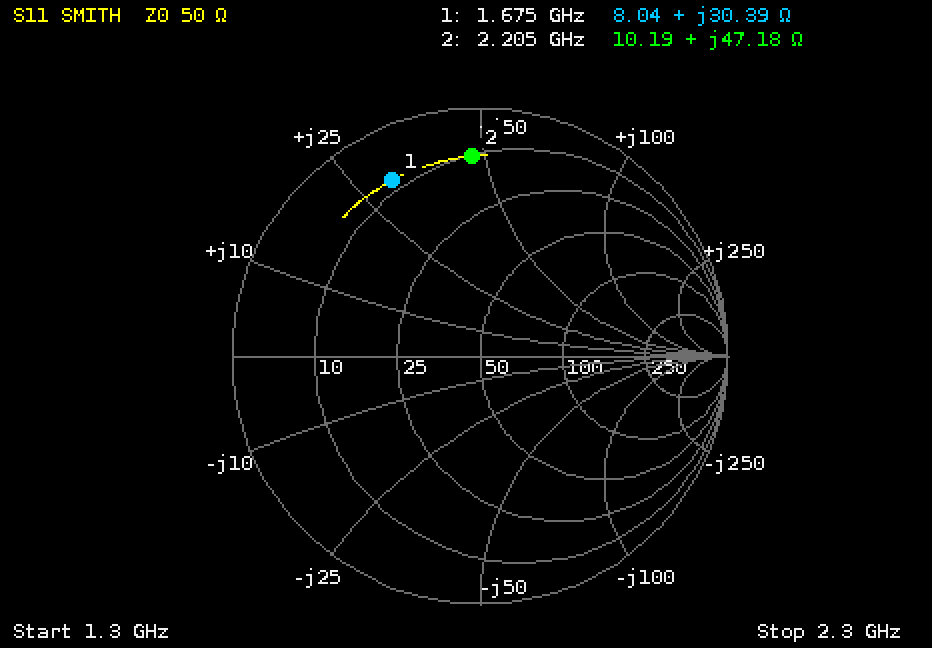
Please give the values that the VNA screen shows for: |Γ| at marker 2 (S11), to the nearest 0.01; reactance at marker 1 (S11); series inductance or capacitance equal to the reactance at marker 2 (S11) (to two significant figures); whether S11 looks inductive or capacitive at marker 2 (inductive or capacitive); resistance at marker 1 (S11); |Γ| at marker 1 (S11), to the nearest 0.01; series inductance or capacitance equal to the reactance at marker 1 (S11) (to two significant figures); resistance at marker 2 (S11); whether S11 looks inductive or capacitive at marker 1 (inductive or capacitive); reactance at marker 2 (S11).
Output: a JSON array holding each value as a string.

["0.81", "+30.39 Ω", "3.4 nH", "inductive", "8.04 Ω", "0.79", "2.9 nH", "10.19 Ω", "inductive", "+47.18 Ω"]
